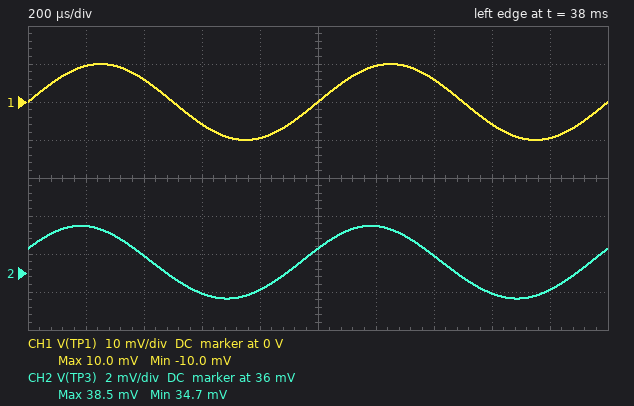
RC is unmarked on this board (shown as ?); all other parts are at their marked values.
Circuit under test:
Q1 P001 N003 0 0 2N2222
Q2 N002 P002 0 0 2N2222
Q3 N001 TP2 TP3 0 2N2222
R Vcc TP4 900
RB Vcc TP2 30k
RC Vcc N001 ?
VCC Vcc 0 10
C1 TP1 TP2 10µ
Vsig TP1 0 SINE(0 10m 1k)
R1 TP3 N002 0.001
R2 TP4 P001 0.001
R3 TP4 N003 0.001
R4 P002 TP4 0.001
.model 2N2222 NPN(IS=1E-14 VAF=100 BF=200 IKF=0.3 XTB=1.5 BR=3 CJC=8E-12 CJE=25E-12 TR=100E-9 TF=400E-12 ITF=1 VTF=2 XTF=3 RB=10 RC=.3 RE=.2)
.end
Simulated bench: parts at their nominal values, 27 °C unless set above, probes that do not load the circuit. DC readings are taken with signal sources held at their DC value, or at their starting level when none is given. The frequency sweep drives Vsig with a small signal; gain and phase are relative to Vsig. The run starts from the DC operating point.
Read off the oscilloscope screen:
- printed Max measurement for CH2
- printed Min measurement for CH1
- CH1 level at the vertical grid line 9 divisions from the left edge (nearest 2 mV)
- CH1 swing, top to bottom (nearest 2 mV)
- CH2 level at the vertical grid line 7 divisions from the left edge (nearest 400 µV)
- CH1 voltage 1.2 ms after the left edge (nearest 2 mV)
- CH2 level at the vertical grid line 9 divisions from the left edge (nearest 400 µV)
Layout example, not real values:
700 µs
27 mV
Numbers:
38.5 mV
-10.0 mV
-10 mV
20 mV
36.8 mV
10 mV
35.2 mV
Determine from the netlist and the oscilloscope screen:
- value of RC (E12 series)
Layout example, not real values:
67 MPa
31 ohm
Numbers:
2.2 kΩ
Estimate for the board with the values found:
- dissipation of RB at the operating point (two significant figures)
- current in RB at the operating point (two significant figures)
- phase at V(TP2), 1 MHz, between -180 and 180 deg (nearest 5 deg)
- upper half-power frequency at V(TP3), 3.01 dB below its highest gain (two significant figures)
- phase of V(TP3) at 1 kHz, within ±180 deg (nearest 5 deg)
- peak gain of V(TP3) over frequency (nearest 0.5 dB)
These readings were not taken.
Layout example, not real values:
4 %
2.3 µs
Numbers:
2.9 mW
310 µA
0 deg
460 MHz
25 deg
-13.0 dB
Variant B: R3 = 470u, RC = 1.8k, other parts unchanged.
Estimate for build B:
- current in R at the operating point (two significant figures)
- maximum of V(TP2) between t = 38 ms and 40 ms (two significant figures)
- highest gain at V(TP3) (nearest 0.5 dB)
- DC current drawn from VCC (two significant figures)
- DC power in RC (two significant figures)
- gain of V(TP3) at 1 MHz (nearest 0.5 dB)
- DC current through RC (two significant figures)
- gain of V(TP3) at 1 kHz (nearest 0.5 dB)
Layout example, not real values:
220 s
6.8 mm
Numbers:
10 mA
760 mV
-11.5 dB
16 mA
54 mW
-12.0 dB
5.5 mA
-13.0 dB
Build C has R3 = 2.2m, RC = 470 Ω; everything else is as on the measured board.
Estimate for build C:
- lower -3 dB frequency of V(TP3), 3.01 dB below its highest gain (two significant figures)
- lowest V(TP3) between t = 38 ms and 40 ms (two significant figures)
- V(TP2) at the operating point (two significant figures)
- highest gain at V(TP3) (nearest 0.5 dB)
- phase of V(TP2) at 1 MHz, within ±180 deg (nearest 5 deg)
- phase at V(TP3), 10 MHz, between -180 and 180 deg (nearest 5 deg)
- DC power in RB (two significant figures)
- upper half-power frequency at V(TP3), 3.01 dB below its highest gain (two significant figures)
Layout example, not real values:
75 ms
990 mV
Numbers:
22 Hz
5.0 V
5.7 V
0 dB
0 deg
0 deg
620 µW
3.2 GHz
